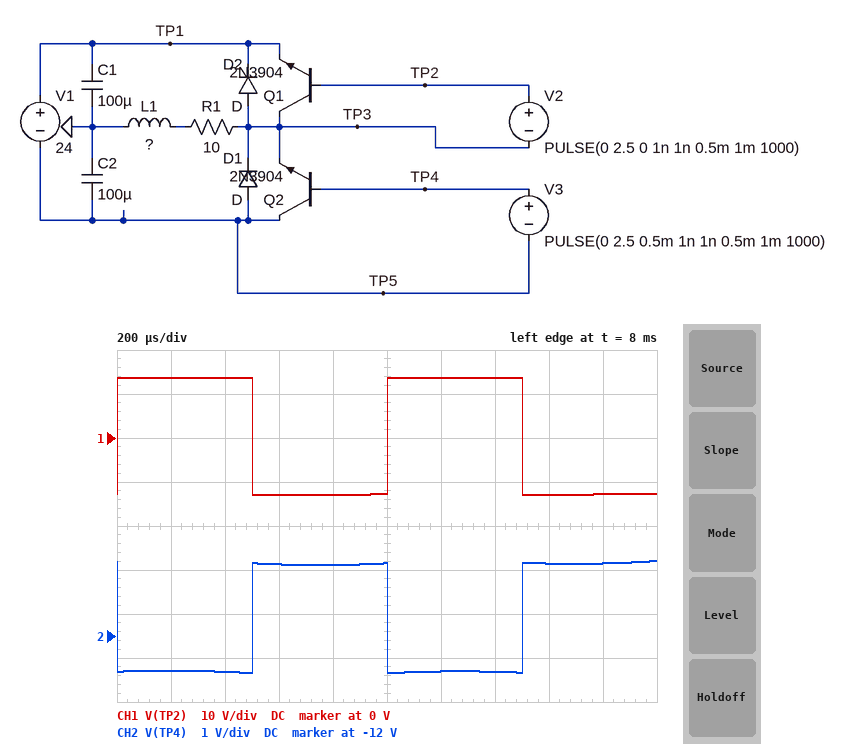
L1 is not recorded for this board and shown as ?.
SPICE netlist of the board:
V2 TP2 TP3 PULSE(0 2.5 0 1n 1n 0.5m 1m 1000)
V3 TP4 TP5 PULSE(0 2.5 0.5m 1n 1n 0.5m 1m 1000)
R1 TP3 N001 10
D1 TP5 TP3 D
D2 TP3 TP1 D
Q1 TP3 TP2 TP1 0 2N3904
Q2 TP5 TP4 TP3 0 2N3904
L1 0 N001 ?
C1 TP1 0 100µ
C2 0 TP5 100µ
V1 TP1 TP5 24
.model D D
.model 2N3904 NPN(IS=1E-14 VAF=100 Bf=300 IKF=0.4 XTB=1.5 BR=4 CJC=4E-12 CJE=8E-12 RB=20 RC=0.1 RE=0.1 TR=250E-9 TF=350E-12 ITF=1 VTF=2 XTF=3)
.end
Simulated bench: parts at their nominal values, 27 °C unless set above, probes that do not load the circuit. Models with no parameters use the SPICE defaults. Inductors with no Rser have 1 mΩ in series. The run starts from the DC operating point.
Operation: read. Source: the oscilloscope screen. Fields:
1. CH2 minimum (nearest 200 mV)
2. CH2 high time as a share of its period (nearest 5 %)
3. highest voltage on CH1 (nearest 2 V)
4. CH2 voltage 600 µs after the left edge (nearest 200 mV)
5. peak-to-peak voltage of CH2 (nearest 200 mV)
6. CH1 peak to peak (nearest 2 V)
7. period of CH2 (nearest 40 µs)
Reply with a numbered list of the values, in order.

1. -12.8 V
2. 50 %
3. 14 V
4. -10.4 V
5. 2.6 V
6. 26 V
7. 1.00 ms
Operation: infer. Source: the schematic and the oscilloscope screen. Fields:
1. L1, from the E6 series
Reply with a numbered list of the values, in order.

1. 47 mH
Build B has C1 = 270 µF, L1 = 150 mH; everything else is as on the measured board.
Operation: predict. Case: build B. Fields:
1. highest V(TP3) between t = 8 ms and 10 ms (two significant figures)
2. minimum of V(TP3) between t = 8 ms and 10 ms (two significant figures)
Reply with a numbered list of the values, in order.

1. 13 V
2. -11 V
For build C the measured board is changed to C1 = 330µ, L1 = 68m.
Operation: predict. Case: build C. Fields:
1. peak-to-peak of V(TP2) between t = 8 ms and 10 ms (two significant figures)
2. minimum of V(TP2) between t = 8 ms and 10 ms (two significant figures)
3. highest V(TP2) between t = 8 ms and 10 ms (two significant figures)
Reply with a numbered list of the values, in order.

1. 27 V
2. -12 V
3. 15 V
